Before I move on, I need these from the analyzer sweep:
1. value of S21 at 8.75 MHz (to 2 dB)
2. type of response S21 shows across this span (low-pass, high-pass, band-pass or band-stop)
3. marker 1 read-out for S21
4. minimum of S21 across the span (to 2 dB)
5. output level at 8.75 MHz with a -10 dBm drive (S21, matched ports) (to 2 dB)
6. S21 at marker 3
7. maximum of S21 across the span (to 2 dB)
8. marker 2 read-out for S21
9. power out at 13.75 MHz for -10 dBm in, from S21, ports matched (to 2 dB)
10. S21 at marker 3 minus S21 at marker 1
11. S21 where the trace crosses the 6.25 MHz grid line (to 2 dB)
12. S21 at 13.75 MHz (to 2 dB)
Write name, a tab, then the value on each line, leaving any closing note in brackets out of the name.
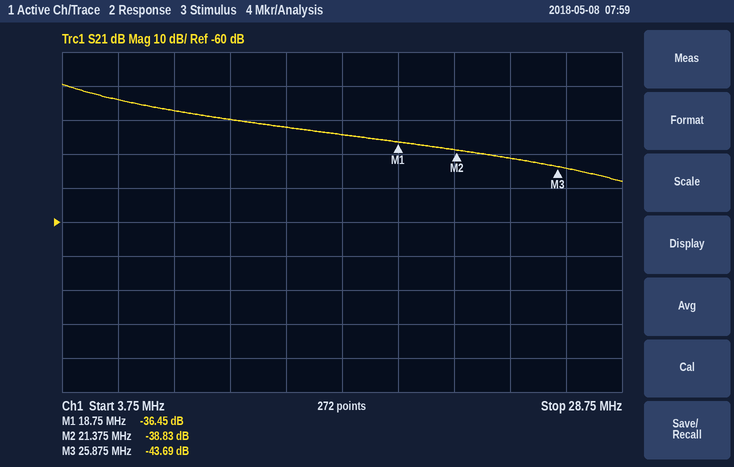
value of S21 at 8.75 MHz	-28 dB
type of response S21 shows across this span	low-pass
marker 1 read-out for S21	-36.45 dB
minimum of S21 across the span	-48 dB
output level at 8.75 MHz with a -10 dBm drive (S21, matched ports)	-38 dBm
S21 at marker 3	-43.69 dB
maximum of S21 across the span	-20 dB
marker 2 read-out for S21	-38.83 dB
power out at 13.75 MHz for -10 dBm in, from S21, ports matched	-42 dBm
S21 at marker 3 minus S21 at marker 1	-7.24 dB
S21 where the trace crosses the 6.25 MHz grid line	-24 dB
S21 at 13.75 MHz	-32 dB
